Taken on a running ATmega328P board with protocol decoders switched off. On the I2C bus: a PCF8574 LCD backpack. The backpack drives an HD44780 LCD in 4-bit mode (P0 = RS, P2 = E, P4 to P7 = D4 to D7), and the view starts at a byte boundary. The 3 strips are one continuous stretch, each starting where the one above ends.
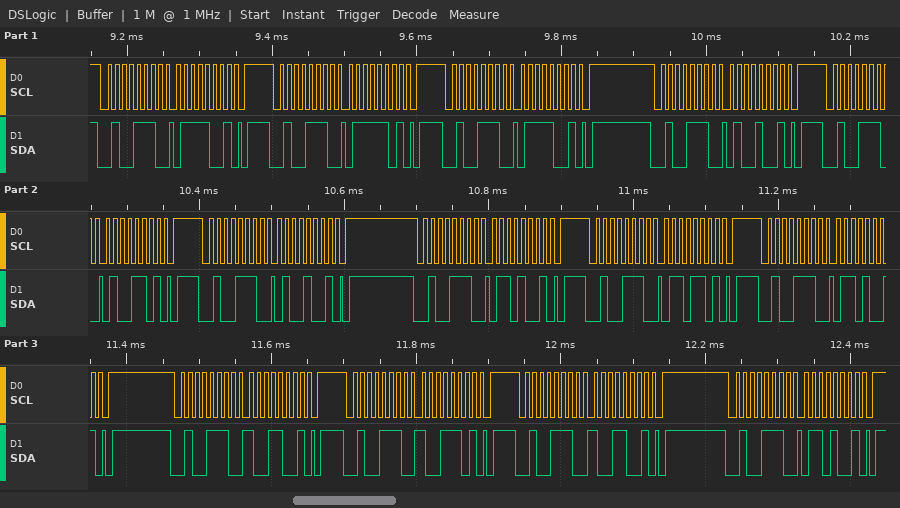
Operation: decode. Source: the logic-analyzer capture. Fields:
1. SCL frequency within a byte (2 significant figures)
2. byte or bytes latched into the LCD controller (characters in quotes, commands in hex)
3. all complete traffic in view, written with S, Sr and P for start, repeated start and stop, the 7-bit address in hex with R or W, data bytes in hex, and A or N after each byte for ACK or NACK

100 kHz
't' 'i'
S 27W A 79 A P S 27W A 7D A P S 27W A 79 A P S 27W A 49 A P S 27W A 4D A P S 27W A 49 A P S 27W A 69 A P S 27W A 6D A P S 27W A 69 A P S 27W A 99 A P S 27W A 9D A P S 27W A 99 A P S 27W A 69 A P
